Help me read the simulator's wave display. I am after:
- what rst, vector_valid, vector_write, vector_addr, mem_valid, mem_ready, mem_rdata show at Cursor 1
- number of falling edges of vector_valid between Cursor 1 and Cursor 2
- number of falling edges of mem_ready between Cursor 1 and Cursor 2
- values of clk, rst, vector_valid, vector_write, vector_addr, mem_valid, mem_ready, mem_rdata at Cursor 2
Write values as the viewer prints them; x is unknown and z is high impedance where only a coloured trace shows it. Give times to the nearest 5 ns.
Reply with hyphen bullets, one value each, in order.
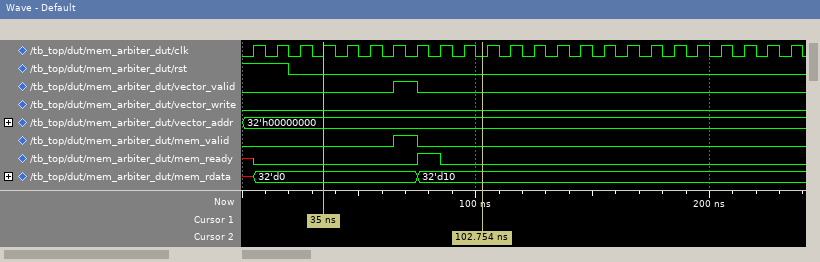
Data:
- rst=0, vector_valid=0, vector_write=0, vector_addr=32'h00000000, mem_valid=0, mem_ready=0, mem_rdata=32'd0
- 1
- 1
- clk=0, rst=0, vector_valid=0, vector_write=0, vector_addr=32'h00000000, mem_valid=0, mem_ready=0, mem_rdata=32'd10
